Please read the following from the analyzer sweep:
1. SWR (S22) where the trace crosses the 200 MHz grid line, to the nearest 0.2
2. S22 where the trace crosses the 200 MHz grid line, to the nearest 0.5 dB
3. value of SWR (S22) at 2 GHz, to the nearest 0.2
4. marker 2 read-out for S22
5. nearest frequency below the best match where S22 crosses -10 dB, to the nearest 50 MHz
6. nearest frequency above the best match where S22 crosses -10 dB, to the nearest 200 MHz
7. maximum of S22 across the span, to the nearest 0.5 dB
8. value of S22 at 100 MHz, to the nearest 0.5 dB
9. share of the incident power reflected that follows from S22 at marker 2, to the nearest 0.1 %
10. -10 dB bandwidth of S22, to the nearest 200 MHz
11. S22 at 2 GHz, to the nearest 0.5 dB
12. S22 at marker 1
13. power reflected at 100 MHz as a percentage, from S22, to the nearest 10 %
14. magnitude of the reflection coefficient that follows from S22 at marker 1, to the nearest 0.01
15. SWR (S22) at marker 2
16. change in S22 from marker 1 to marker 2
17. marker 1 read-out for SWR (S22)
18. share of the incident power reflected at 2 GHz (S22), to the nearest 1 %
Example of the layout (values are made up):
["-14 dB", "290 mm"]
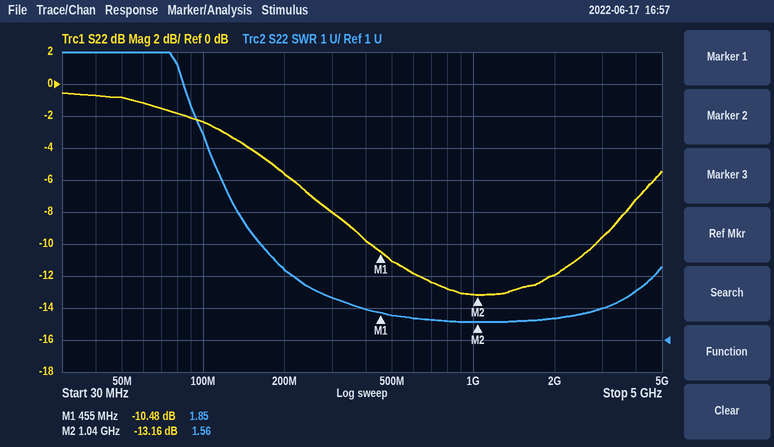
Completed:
["3.2", "-5.5 dB", "1.6", "-13.16 dB", "400 MHz", "2.8 GHz", "-0.5 dB", "-2.5 dB", "4.8 %", "2.4 GHz", "-12.0 dB", "-10.48 dB", "60 %", "0.30", "1.56", "-2.68 dB", "1.85", "6 %"]
